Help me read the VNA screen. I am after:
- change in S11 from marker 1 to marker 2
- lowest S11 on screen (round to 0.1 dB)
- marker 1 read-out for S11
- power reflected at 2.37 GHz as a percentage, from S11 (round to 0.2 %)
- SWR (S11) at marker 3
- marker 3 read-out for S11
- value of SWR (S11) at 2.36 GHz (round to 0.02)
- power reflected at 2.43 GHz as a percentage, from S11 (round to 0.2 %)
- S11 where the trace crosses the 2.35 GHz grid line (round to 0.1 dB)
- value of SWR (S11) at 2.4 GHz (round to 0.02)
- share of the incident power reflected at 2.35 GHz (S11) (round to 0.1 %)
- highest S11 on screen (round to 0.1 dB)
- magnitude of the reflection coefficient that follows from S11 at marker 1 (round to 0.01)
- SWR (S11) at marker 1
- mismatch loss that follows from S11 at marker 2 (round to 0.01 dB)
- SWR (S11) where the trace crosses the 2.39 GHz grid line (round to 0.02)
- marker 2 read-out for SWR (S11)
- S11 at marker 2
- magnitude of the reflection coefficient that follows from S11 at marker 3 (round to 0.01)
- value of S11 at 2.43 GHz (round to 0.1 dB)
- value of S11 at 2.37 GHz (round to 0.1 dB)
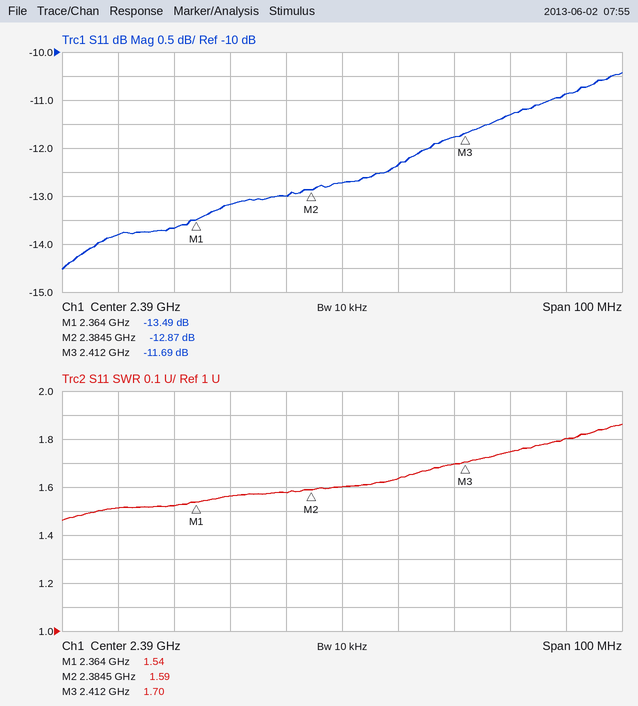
0.62 dB
-14.5 dB
-13.49 dB
4.8 %
1.70
-11.69 dB
1.52
8.2 %
-13.8 dB
1.64
4.2 %
-10.4 dB
0.21
1.54
0.23 dB
1.60
1.59
-12.87 dB
0.26
-10.9 dB
-13.2 dB
